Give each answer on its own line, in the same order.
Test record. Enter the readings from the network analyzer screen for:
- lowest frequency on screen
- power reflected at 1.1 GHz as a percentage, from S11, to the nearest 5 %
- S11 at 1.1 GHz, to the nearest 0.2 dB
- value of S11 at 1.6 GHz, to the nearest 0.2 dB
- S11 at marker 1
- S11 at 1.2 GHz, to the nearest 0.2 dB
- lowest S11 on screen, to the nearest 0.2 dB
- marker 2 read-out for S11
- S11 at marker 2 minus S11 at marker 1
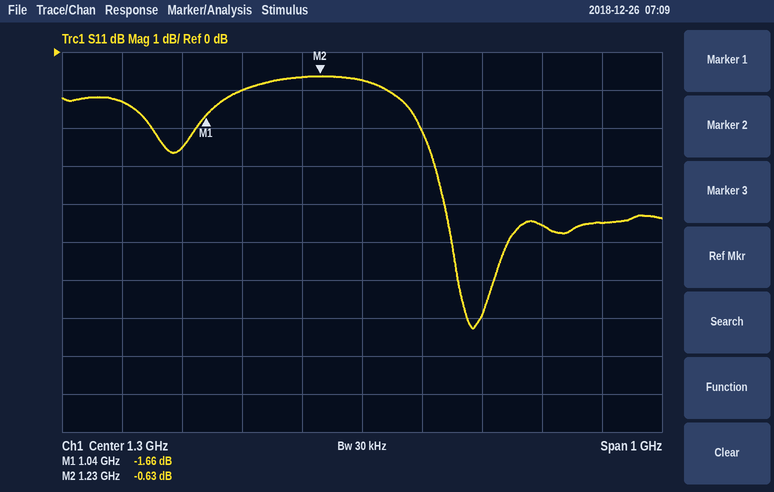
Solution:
800 MHz
80 %
-1.0 dB
-4.6 dB
-1.66 dB
-0.6 dB
-7.2 dB
-0.63 dB
1.03 dB
